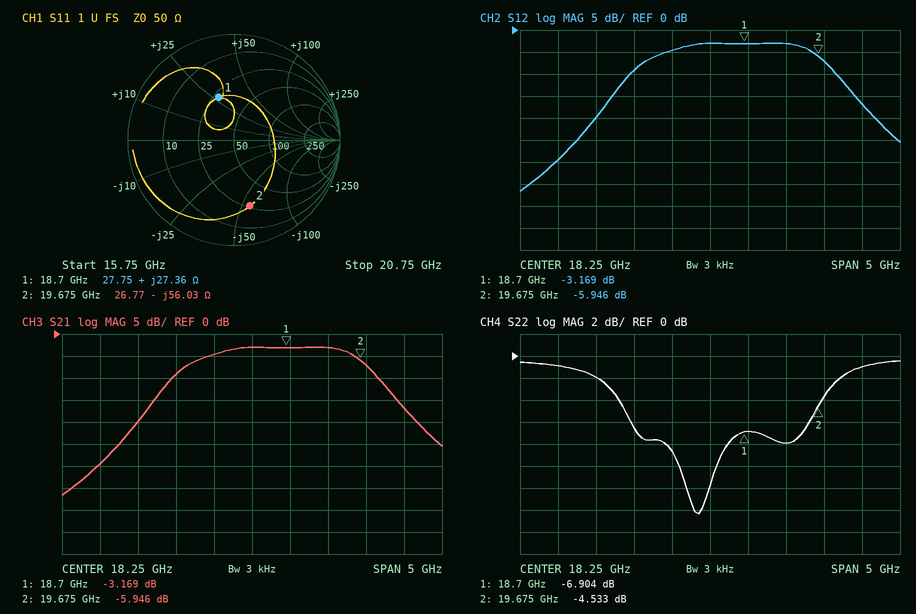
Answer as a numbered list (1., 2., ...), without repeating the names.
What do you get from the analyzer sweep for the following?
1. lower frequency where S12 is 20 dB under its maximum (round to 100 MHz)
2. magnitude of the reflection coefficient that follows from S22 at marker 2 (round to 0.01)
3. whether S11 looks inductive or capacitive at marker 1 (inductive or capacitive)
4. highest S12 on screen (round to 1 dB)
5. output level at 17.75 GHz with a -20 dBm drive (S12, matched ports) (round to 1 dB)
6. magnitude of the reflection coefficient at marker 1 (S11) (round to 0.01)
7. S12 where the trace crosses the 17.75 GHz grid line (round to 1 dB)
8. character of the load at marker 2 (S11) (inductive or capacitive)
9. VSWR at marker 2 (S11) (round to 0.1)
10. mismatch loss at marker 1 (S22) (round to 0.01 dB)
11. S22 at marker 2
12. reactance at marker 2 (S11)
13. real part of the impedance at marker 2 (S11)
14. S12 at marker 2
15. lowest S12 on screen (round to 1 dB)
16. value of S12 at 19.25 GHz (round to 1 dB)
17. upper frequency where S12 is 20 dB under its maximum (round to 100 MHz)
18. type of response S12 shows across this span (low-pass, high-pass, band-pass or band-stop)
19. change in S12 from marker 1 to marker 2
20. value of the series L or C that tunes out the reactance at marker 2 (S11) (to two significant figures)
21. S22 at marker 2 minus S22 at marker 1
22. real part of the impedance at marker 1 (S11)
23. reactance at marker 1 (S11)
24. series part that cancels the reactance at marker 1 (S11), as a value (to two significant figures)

1. 16.6 GHz
2. 0.59
3. inductive
4. -3 dB
5. -25 dBm
6. 0.43
7. -5 dB
8. capacitive
9. 4.5
10. 0.99 dB
11. -4.533 dB
12. -56.03 Ω
13. 26.77 Ω
14. -5.946 dB
15. -37 dB
16. -3 dB
17. 20.6 GHz
18. band-pass
19. -2.777 dB
20. 450 pH
21. 2.371 dB
22. 27.75 Ω
23. +27.36 Ω
24. 310 fF
